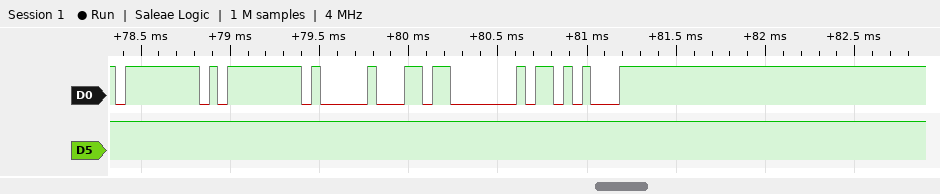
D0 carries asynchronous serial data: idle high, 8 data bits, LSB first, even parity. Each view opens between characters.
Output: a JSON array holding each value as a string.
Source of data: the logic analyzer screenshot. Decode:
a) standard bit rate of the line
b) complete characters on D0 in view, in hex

["19200 baud", "FF, FF, 10, 03, 2B"]
